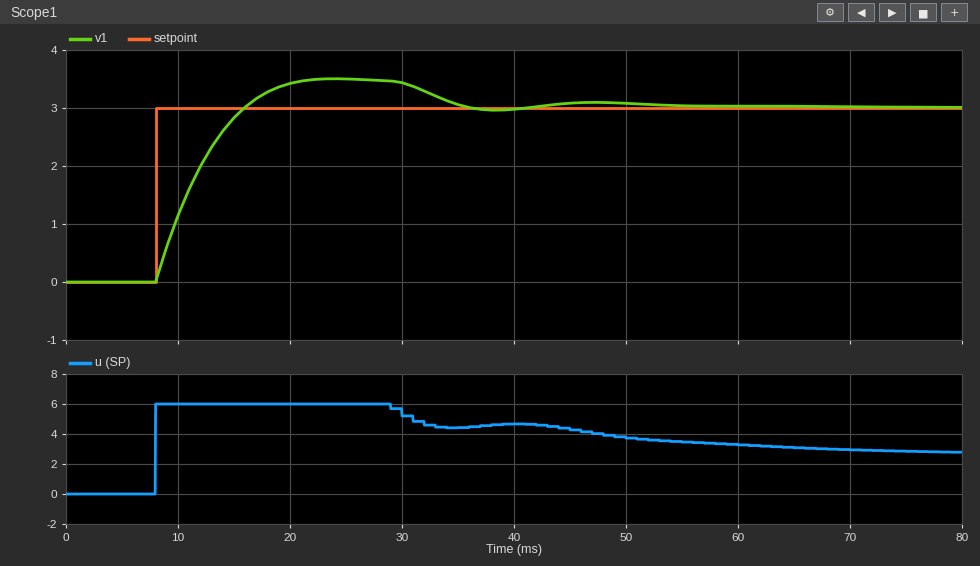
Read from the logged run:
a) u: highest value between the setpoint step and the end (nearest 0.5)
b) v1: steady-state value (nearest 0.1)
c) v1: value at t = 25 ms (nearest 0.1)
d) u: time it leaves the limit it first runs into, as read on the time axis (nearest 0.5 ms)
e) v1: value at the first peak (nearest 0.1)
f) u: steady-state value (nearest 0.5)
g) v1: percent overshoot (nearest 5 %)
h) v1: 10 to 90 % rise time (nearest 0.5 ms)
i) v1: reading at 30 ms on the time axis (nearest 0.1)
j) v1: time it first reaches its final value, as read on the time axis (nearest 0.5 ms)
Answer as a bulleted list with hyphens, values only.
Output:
- 6.0
- 3.0
- 3.5
- 29.0 ms
- 3.5
- 3.0
- 15 %
- 6.0 ms
- 3.4
- 16.0 ms
